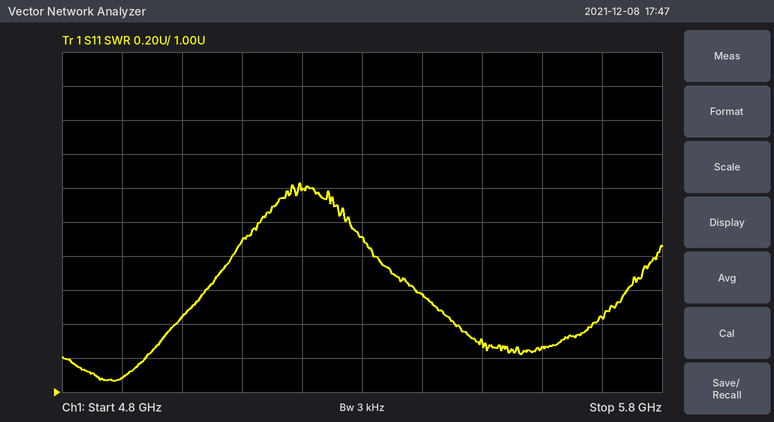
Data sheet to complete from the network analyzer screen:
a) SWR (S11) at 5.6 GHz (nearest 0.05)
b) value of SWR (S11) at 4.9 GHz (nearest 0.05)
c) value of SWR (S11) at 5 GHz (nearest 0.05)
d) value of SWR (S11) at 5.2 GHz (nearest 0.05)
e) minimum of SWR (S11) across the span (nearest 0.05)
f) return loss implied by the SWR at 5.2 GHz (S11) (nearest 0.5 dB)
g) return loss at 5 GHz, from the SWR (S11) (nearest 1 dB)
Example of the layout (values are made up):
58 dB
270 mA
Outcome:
1.25
1.10
1.45
2.20
1.05
8.5 dB
15 dB
